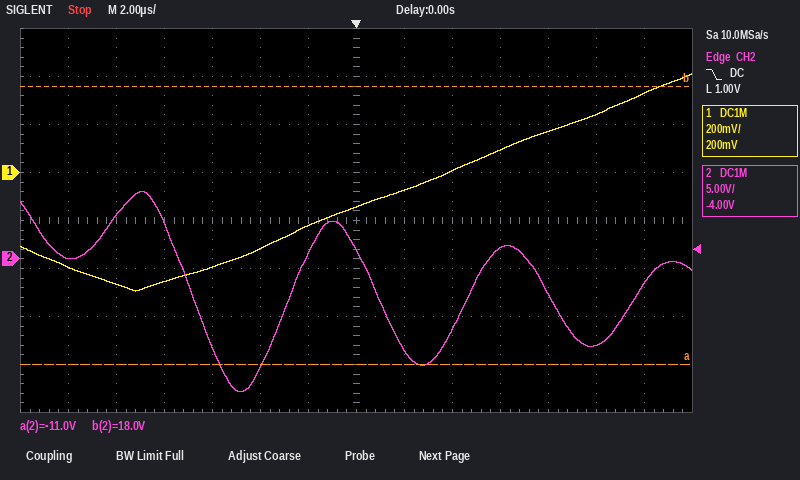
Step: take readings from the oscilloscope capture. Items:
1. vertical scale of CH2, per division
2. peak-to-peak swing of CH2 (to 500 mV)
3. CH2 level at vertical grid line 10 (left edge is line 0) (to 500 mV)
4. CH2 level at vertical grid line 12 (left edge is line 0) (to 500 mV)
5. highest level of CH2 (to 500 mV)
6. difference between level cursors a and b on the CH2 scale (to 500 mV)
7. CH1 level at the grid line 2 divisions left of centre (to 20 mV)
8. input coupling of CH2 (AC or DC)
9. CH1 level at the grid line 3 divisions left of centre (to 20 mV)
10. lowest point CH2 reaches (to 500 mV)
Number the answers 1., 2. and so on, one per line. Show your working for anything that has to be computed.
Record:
1. 5 V
2. 7.0 V − (-14.0 V) = 21.0 V
3. 1.0 V
4. -9.0 V
5. 7.0 V
6. 29.0 V
7. -320 mV
8. DC
9. -400 mV
10. -14.0 V
